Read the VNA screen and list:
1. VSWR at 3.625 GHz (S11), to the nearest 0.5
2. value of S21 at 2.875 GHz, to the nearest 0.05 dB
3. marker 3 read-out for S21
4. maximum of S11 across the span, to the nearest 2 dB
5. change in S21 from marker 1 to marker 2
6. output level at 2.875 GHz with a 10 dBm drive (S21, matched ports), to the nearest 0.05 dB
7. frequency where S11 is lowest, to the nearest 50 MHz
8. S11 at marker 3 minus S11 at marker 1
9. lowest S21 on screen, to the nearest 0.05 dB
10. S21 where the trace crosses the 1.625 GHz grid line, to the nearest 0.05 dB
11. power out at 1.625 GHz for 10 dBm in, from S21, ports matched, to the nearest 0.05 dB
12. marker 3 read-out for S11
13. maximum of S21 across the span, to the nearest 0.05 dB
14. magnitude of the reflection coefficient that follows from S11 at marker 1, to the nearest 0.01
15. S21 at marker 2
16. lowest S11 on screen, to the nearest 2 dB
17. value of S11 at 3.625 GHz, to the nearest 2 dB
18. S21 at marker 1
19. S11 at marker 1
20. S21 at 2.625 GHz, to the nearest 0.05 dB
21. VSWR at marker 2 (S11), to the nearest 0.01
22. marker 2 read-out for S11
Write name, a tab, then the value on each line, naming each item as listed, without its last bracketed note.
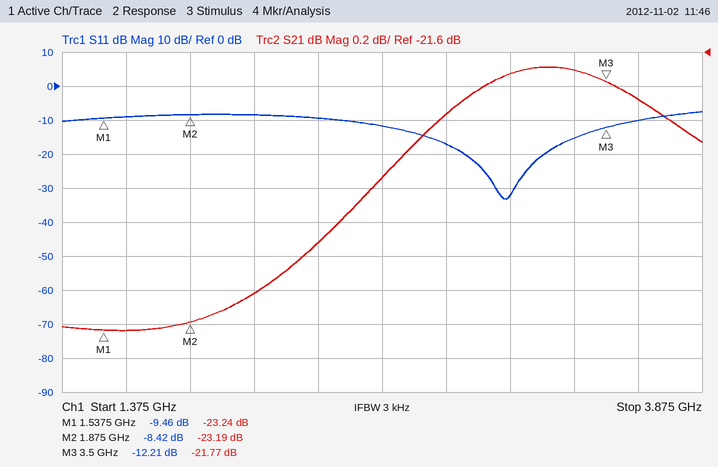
VSWR at 3.625 GHz (S11), to the nearest 0.5	2.0
value of S21 at 2.875 GHz, to the nearest 0.05 dB	-21.95 dB
marker 3 read-out for S21	-21.77 dB
maximum of S11 across the span, to the nearest 2 dB	-8 dB
change in S21 from marker 1 to marker 2	0.05 dB
output level at 2.875 GHz with a 10 dBm drive (S21, matched ports), to the nearest 0.05 dB	-11.95 dBm
frequency where S11 is lowest, to the nearest 50 MHz	3.10 GHz
S11 at marker 3 minus S11 at marker 1	-2.75 dB
lowest S21 on screen, to the nearest 0.05 dB	-23.25 dB
S21 where the trace crosses the 1.625 GHz grid line, to the nearest 0.05 dB	-23.25 dB
power out at 1.625 GHz for 10 dBm in, from S21, ports matched, to the nearest 0.05 dB	-13.25 dBm
marker 3 read-out for S11	-12.21 dB
maximum of S21 across the span, to the nearest 0.05 dB	-21.70 dB
magnitude of the reflection coefficient that follows from S11 at marker 1, to the nearest 0.01	0.34
S21 at marker 2	-23.19 dB
lowest S11 on screen, to the nearest 2 dB	-34 dB
value of S11 at 3.625 GHz, to the nearest 2 dB	-10 dB
S21 at marker 1	-23.24 dB
S11 at marker 1	-9.46 dB
S21 at 2.625 GHz, to the nearest 0.05 dB	-22.35 dB
VSWR at marker 2 (S11), to the nearest 0.01	2.22
marker 2 read-out for S11	-8.42 dB
